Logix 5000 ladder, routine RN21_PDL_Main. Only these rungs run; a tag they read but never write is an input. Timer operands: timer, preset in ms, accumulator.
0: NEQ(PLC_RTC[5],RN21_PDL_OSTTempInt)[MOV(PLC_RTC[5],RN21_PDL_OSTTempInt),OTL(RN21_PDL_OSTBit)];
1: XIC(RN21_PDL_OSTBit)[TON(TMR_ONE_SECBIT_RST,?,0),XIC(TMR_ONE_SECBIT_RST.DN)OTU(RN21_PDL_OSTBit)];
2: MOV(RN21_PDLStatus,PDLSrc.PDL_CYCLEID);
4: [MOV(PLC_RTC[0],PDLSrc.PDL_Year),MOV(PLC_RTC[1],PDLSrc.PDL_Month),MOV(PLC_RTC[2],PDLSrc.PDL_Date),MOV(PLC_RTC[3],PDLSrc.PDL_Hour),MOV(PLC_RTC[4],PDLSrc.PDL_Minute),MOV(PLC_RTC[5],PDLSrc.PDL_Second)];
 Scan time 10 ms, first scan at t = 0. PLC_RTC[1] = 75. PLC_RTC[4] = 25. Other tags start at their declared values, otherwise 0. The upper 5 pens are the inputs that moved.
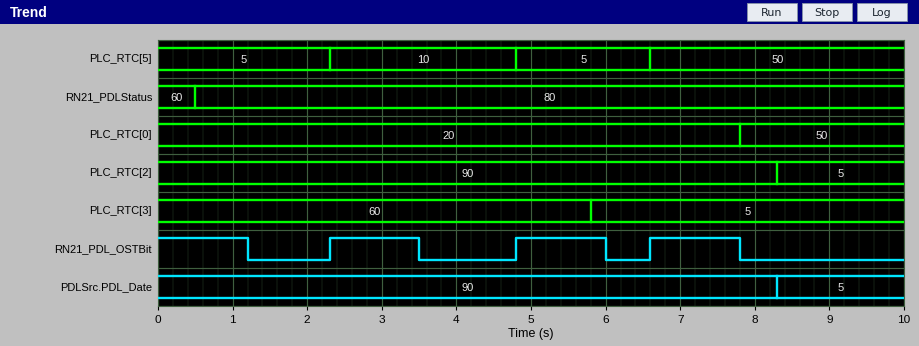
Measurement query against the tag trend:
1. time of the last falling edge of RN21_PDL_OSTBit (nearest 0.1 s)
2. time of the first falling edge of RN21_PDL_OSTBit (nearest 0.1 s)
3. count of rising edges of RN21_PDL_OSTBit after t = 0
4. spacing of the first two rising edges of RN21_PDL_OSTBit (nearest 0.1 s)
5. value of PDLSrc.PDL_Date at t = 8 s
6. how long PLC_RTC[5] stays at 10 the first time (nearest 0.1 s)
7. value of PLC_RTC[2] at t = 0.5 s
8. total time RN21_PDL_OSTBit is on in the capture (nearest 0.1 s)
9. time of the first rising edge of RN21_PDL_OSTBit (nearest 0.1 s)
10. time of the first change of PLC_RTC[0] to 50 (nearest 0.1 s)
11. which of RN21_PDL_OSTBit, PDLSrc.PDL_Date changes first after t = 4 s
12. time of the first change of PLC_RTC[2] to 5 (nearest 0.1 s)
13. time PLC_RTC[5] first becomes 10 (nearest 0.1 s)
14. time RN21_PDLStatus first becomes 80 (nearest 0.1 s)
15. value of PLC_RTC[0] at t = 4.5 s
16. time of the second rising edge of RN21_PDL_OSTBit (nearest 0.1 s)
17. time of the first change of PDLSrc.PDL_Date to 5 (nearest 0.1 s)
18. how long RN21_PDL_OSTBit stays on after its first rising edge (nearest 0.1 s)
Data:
7.8 s
1.2 s
3
2.5 s
90
2.5 s
90
4.8 s
2.3 s
7.8 s
RN21_PDL_OSTBit
8.3 s
2.3 s
0.5 s
20
4.8 s
8.3 s
1.2 s
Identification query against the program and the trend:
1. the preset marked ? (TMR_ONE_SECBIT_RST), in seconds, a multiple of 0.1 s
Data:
1.2 s
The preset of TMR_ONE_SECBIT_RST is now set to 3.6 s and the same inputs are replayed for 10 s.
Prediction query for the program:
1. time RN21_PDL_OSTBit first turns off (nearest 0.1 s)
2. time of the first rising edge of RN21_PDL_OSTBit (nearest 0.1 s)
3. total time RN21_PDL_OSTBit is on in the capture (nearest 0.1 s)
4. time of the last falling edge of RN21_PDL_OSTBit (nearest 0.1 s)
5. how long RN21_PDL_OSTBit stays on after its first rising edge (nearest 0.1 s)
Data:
3.6 s
4.8 s
7.2 s
8.4 s
3.6 s
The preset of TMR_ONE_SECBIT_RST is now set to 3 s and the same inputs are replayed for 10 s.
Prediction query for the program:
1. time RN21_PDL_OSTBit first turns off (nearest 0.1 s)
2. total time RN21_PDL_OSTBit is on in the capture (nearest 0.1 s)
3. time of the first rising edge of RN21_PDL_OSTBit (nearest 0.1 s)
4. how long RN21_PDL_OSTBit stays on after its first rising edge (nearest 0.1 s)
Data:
3.0 s
6.0 s
4.8 s
3.0 s
